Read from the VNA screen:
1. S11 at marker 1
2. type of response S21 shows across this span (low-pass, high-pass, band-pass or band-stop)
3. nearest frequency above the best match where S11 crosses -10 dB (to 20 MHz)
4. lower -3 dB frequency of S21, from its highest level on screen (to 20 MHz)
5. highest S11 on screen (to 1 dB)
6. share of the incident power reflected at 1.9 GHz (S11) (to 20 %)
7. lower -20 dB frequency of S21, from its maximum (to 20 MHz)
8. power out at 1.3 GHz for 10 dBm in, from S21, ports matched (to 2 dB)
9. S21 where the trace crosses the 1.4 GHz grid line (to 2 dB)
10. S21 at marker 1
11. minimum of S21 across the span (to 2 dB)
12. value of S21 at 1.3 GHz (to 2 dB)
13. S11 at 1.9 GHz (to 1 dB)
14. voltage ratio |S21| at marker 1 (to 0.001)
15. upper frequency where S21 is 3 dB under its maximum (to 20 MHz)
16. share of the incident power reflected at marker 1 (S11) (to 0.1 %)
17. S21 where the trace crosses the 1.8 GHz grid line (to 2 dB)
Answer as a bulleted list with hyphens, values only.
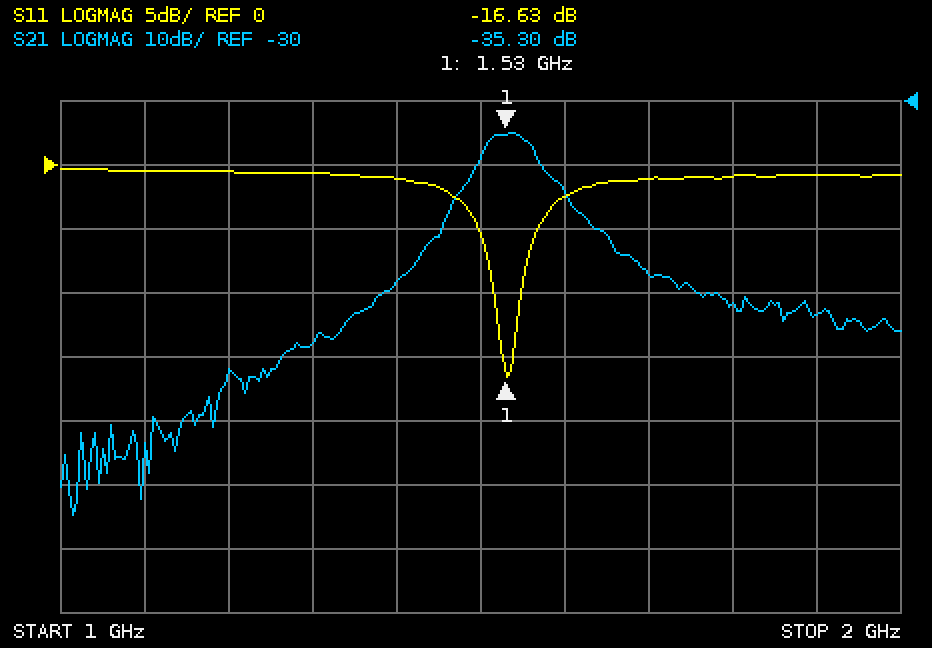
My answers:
- -16.63 dB
- band-pass
- 1.54 GHz
- 1.50 GHz
- 0 dB
- 80 %
- 1.42 GHz
- -58 dBm
- -58 dB
- -35.30 dB
- -94 dB
- -68 dB
- -1 dB
- 0.017
- 1.56 GHz
- 2.2 %
- -62 dB
